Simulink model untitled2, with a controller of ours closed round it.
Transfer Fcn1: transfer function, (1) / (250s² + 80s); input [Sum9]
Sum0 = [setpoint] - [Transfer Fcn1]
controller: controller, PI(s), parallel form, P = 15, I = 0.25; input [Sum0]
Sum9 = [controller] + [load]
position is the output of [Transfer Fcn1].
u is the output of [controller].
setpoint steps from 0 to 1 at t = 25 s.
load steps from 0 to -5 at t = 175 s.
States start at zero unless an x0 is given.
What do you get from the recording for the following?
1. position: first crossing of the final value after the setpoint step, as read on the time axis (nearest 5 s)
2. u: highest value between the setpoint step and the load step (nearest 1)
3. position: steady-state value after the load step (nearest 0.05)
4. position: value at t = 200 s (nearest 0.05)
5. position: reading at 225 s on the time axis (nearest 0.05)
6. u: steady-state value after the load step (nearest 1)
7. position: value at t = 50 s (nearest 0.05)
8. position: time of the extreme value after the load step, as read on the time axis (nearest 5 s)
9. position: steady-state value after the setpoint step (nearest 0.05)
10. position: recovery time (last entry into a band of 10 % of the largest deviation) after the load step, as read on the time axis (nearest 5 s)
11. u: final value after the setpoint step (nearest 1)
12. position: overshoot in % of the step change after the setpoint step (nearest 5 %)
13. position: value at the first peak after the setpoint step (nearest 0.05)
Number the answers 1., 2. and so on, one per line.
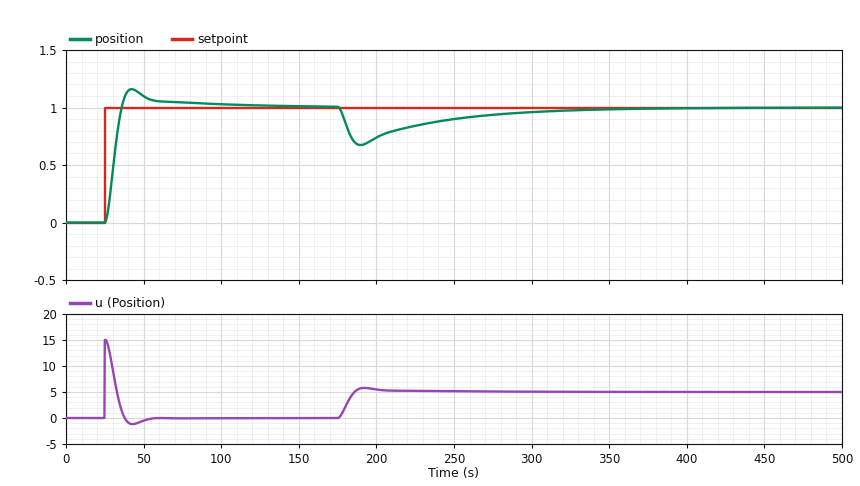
1. 35 s
2. 15
3. 1.00
4. 0.75
5. 0.85
6. 5
7. 1.10
8. 190 s
9. 1.00
10. 310 s
11. 0
12. 15 %
13. 1.15
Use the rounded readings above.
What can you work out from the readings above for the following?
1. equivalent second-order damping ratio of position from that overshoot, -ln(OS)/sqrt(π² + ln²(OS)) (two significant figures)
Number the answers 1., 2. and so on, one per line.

1. 0.52
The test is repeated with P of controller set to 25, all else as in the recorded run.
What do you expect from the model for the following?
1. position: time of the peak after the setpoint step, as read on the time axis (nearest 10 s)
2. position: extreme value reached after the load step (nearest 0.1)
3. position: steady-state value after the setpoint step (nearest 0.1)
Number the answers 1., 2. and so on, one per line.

1. 40 s
2. 0.8
3. 1.0
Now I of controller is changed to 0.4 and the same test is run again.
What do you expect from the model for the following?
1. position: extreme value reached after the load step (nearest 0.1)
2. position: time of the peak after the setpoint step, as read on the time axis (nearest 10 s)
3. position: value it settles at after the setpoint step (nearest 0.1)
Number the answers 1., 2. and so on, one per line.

1. 0.7
2. 40 s
3. 1.0
